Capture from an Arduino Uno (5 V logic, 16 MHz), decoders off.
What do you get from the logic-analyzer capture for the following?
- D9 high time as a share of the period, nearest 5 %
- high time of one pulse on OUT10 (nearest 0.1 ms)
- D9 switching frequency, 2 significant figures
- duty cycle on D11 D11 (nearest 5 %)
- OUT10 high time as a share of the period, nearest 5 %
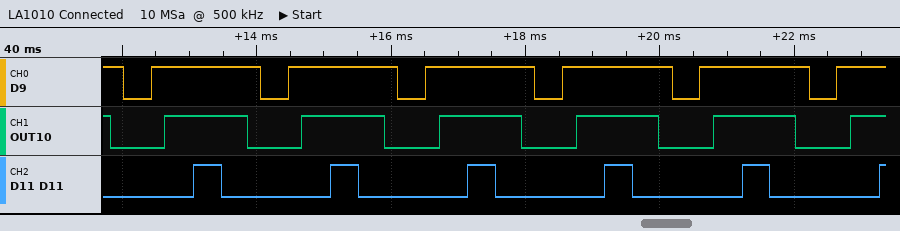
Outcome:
80 %
1.2 ms
490 Hz
20 %
60 %
